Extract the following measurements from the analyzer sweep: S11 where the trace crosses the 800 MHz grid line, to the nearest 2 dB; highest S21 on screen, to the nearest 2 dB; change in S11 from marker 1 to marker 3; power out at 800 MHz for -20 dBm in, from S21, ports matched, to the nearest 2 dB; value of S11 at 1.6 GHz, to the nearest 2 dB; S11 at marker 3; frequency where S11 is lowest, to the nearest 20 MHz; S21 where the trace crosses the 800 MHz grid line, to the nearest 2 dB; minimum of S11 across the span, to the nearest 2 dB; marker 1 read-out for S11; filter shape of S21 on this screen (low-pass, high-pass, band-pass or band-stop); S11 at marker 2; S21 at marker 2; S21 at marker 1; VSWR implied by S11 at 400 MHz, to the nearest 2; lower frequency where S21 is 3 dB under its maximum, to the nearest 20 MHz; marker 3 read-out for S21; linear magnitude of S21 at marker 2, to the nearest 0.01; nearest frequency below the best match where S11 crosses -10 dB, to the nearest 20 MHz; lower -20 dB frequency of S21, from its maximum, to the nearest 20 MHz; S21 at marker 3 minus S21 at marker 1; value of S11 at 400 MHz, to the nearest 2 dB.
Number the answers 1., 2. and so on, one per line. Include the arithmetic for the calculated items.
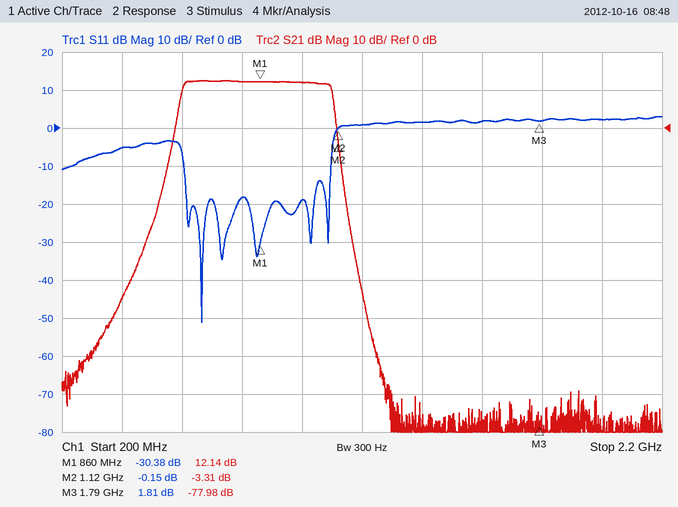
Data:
1. -18 dB
2. 12 dB
3. 1.81 − (-30.38) = 32.19 dB
4. -20 dBm + (12 dB) = -8 dBm
5. 2 dB
6. 1.81 dB
7. 660 MHz
8. 12 dB
9. -52 dB
10. -30.38 dB
11. band-pass
12. -0.15 dB
13. -3.31 dB
14. 12.14 dB
15. |Γ| = 10^(-6/20) = 0.5012; VSWR = (1 + 0.5012)/(1 − 0.5012) ≈ 3.01, so 4 to the nearest 2
16. 600 MHz
17. -77.98 dB
18. 10^(-3.31/20) ≈ 0.68
19. 600 MHz
20. 560 MHz
21. -77.98 − (12.14) = -90.12 dB
22. -6 dB
